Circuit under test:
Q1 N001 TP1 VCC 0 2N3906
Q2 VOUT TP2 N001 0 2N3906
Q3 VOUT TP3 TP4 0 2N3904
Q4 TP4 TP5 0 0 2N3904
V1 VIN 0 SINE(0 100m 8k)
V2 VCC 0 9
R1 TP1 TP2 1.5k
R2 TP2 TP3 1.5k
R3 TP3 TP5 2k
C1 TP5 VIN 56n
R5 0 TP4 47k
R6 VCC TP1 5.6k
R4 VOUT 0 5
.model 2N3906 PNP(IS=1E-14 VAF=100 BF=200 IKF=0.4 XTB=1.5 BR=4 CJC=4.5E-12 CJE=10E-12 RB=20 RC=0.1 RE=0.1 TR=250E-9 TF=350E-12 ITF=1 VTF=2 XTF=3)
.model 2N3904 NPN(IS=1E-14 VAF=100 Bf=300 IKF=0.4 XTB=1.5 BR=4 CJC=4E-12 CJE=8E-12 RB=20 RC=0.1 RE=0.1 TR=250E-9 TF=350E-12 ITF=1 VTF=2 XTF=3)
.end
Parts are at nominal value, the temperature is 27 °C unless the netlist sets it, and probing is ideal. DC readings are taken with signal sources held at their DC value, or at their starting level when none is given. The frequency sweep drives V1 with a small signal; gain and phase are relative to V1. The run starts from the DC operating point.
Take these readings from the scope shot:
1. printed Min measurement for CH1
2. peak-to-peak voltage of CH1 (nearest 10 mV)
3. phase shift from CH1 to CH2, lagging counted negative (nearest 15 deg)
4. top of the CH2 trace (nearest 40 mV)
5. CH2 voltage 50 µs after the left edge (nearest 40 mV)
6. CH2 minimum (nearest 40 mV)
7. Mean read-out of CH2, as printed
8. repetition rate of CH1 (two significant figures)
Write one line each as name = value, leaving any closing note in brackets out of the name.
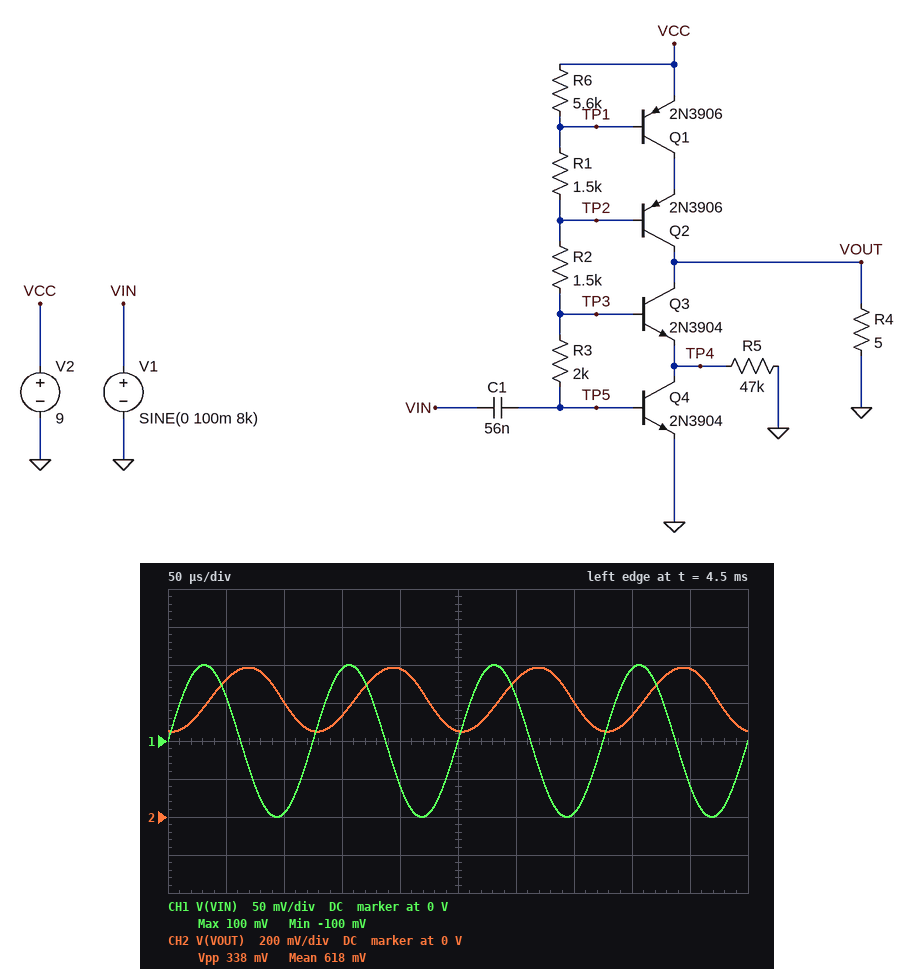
printed Min measurement for CH1 = -100 mV
peak-to-peak voltage of CH1 = 200 mV
phase shift from CH1 to CH2, lagging counted negative = -105 deg
top of the CH2 trace = 800 mV
CH2 voltage 50 µs after the left edge = 720 mV
CH2 minimum = 440 mV
Mean read-out of CH2, as printed = 618 mV
repetition rate of CH1 = 8.0 kHz
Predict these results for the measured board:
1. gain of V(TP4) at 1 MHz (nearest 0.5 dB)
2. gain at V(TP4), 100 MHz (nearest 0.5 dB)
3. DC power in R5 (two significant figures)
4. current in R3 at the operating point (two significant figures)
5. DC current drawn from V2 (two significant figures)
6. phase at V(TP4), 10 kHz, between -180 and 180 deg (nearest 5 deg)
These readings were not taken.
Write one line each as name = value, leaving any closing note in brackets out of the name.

gain of V(TP4) at 1 MHz = 18.5 dB
gain at V(TP4), 100 MHz = 0.5 dB
DC power in R5 = 6.2 µW
current in R3 at the operating point = 290 µA
DC current drawn from V2 = 200 mA
phase at V(TP4), 10 kHz, between -180 and 180 deg = -105 deg
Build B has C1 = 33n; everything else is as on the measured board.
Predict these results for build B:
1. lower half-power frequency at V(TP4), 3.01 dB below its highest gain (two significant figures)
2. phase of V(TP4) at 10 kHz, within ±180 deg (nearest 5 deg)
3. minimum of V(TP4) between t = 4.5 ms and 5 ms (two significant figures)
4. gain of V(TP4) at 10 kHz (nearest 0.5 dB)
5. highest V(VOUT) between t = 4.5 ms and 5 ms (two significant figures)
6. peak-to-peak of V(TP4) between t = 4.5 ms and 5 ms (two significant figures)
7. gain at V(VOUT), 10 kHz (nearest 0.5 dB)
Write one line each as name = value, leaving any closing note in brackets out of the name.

lower half-power frequency at V(TP4), 3.01 dB below its highest gain = 57 kHz
phase of V(TP4) at 10 kHz, within ±180 deg = -100 deg
minimum of V(TP4) between t = 4.5 ms and 5 ms = 430 mV
gain of V(TP4) at 10 kHz = 3.0 dB
highest V(VOUT) between t = 4.5 ms and 5 ms = 720 mV
peak-to-peak of V(TP4) between t = 4.5 ms and 5 ms = 230 mV
gain at V(VOUT), 10 kHz = 2.0 dB
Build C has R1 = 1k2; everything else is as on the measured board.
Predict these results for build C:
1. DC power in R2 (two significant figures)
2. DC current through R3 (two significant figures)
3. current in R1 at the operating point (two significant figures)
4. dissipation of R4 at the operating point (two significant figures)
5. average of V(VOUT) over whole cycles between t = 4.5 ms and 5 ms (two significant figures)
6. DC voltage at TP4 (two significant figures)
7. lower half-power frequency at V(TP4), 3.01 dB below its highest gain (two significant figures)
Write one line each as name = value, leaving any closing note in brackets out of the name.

DC power in R2 = 15 mW
DC current through R3 = 310 µA
current in R1 at the operating point = 1.7 mA
dissipation of R4 at the operating point = 84 mW
average of V(VOUT) over whole cycles between t = 4.5 ms and 5 ms = 650 mV
DC voltage at TP4 = 570 mV
lower half-power frequency at V(TP4), 3.01 dB below its highest gain = 35 kHz
